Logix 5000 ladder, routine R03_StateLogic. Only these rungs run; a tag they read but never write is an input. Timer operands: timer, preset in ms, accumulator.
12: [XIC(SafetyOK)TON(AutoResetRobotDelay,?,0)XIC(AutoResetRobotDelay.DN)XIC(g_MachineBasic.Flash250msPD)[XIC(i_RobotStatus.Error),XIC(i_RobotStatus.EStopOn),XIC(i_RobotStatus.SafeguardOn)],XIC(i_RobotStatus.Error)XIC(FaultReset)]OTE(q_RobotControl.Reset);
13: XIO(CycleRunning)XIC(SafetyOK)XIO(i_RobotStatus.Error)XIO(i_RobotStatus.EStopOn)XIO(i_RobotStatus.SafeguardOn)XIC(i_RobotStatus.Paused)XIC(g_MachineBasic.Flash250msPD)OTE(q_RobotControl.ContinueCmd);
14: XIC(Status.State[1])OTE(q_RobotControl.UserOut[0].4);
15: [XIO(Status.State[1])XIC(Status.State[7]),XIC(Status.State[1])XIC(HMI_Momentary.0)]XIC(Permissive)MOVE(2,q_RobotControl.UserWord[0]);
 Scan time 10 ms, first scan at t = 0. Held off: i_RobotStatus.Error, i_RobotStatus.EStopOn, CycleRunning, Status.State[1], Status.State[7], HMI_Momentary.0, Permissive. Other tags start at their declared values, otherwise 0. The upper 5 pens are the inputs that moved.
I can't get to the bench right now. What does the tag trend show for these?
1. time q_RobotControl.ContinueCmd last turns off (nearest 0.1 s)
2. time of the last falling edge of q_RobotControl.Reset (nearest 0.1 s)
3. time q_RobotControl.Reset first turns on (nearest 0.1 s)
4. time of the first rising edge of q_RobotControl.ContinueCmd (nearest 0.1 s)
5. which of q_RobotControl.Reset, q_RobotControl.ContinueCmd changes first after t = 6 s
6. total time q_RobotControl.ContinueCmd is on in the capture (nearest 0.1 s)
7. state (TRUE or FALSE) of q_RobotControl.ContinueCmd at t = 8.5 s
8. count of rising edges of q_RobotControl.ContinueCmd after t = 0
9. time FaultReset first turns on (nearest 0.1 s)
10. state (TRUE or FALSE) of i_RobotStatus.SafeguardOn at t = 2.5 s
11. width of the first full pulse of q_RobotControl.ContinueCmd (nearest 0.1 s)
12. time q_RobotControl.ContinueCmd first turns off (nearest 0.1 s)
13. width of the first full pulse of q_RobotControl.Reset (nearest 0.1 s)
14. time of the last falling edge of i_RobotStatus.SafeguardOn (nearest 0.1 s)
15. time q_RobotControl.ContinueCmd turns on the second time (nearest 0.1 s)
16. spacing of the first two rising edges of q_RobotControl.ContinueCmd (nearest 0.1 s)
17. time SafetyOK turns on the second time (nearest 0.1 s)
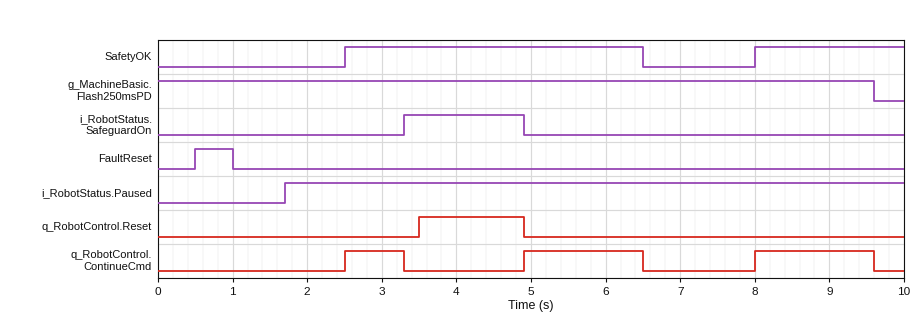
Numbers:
9.6 s
4.9 s
3.5 s
2.5 s
q_RobotControl.ContinueCmd
4.0 s
TRUE
3
0.5 s
FALSE
0.8 s
3.3 s
1.4 s
4.9 s
4.9 s
2.4 s
8.0 s
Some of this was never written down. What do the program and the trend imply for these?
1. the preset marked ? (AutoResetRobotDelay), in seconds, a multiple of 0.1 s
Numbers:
1.0 s
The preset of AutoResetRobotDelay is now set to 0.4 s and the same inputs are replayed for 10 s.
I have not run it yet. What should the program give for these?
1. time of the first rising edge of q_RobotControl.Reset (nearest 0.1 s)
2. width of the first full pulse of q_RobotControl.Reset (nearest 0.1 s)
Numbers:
3.3 s
1.6 s
